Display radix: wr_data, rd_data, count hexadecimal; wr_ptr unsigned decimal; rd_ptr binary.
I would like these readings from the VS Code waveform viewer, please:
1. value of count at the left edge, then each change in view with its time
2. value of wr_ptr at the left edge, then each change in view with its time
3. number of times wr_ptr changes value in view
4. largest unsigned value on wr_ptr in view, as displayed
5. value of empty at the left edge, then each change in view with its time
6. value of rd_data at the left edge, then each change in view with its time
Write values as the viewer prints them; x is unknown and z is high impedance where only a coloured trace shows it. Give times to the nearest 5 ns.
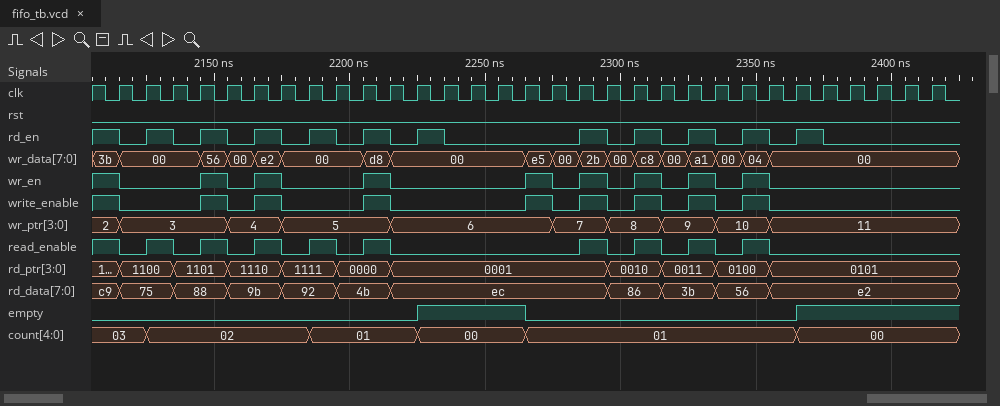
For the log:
03, 02 at 2125 ns, 01 at 2185 ns, 00 at 2225 ns, 01 at 2265 ns, 00 at 2365 ns
2, 3 at 2115 ns, 4 at 2155 ns, 5 at 2175 ns, 6 at 2215 ns, 7 at 2275 ns, 8 at 2295 ns, 9 at 2315 ns, 10 at 2335 ns, 11 at 2355 ns
9
11
0, 1 at 2225 ns, 0 at 2265 ns, 1 at 2365 ns
c9, 75 at 2115 ns, 88 at 2135 ns, 9b at 2155 ns, 92 at 2175 ns, 4b at 2195 ns, ec at 2215 ns, 86 at 2295 ns, 3b at 2315 ns, 56 at 2335 ns, e2 at 2355 ns
